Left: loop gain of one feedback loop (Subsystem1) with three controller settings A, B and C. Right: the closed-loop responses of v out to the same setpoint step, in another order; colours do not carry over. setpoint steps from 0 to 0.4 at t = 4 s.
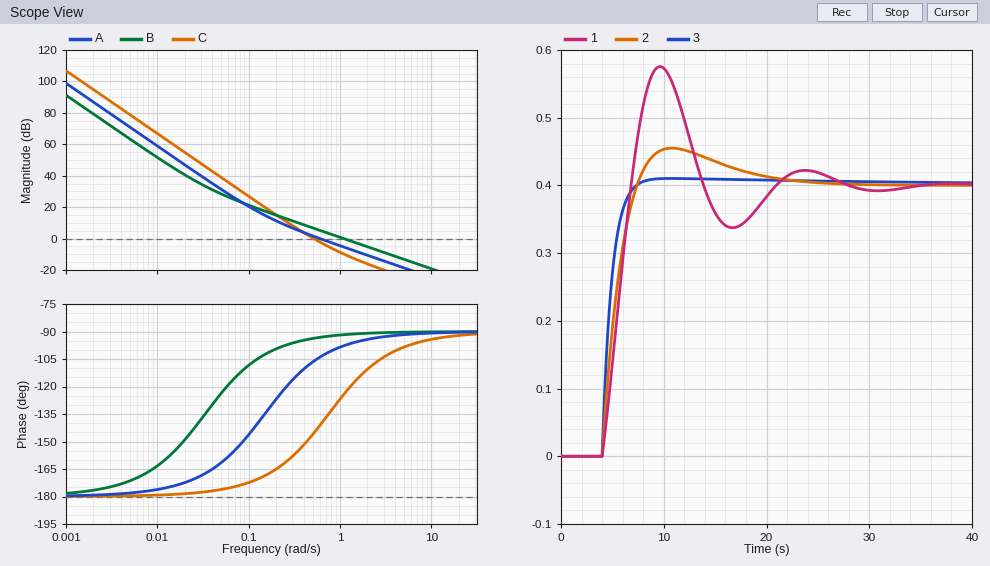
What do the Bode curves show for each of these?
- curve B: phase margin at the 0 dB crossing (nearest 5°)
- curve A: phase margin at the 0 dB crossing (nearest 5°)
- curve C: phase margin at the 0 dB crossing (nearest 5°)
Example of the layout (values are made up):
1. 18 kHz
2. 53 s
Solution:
1. 90°
2. 75°
3. 35°
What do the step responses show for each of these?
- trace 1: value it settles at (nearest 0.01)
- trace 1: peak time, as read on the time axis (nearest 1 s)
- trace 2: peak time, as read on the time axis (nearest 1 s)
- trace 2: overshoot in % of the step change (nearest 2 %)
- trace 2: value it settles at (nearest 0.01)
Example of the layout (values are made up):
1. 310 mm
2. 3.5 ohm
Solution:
1. 0.40
2. 10 s
3. 11 s
4. 14 %
5. 0.40
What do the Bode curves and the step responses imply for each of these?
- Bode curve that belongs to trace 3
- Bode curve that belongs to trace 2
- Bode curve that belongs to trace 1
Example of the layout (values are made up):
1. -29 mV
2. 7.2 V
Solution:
1. B
2. A
3. C
